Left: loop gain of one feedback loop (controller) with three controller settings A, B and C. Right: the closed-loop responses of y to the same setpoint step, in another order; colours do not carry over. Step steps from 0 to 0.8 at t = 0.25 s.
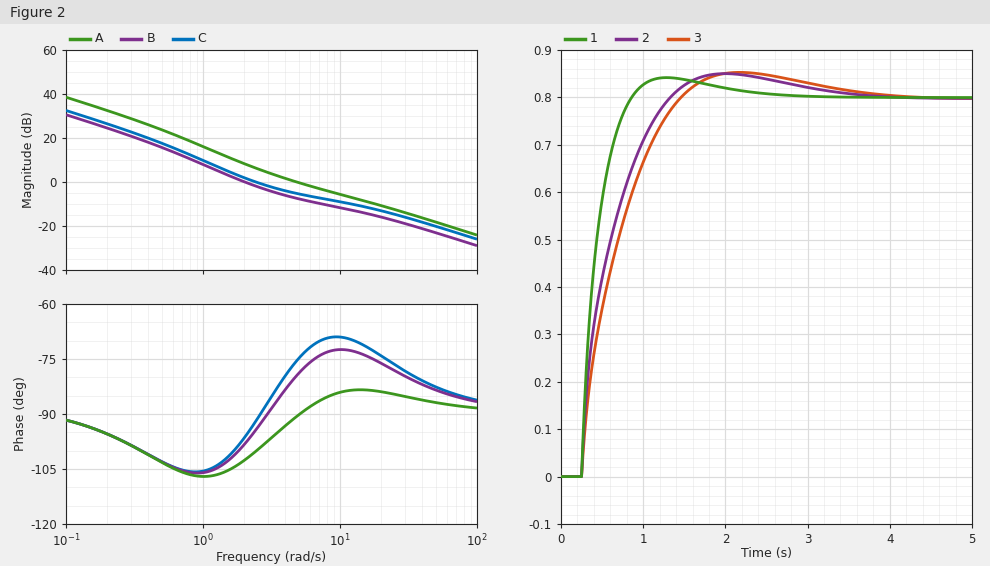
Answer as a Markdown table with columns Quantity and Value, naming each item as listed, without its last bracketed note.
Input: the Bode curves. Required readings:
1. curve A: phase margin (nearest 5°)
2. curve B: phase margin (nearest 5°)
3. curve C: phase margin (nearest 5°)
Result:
| Quantity | Value |
|---|---|
| curve A: phase margin | 90° |
| curve B: phase margin | 80° |
| curve C: phase margin | 90° |
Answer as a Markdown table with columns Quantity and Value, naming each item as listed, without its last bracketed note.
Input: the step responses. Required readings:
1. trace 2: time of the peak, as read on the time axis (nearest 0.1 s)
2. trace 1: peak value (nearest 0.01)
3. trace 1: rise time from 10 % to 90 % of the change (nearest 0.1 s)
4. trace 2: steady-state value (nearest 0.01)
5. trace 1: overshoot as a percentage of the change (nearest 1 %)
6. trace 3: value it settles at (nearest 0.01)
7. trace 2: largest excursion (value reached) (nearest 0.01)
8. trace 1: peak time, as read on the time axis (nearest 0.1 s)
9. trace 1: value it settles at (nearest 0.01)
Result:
| Quantity | Value |
|---|---|
| trace 2: time of the peak, as read on the time axis | 2.0 s |
| trace 1: peak value | 0.84 |
| trace 1: rise time from 10 % to 90 % of the change | 0.4 s |
| trace 2: steady-state value | 0.80 |
| trace 1: overshoot as a percentage of the change | 5 % |
| trace 3: value it settles at | 0.80 |
| trace 2: largest excursion (value reached) | 0.85 |
| trace 1: peak time, as read on the time axis | 1.3 s |
| trace 1: value it settles at | 0.80 |
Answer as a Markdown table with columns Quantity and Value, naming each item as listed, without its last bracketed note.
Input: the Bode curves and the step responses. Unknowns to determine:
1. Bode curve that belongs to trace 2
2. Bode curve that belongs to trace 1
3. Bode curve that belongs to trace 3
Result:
| Quantity | Value |
|---|---|
| Bode curve that belongs to trace 2 | C |
| Bode curve that belongs to trace 1 | A |
| Bode curve that belongs to trace 3 | B |
